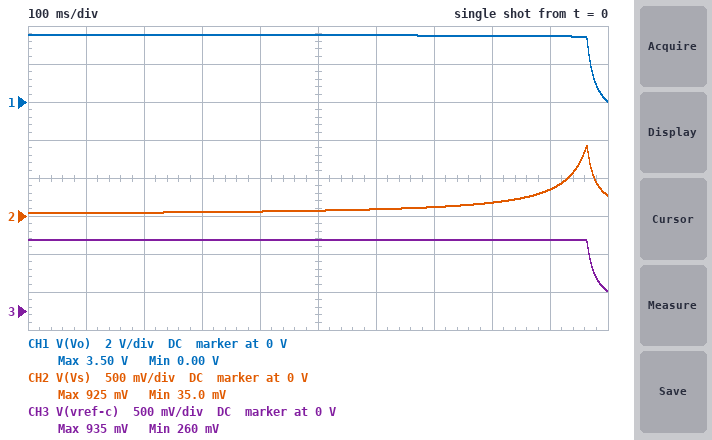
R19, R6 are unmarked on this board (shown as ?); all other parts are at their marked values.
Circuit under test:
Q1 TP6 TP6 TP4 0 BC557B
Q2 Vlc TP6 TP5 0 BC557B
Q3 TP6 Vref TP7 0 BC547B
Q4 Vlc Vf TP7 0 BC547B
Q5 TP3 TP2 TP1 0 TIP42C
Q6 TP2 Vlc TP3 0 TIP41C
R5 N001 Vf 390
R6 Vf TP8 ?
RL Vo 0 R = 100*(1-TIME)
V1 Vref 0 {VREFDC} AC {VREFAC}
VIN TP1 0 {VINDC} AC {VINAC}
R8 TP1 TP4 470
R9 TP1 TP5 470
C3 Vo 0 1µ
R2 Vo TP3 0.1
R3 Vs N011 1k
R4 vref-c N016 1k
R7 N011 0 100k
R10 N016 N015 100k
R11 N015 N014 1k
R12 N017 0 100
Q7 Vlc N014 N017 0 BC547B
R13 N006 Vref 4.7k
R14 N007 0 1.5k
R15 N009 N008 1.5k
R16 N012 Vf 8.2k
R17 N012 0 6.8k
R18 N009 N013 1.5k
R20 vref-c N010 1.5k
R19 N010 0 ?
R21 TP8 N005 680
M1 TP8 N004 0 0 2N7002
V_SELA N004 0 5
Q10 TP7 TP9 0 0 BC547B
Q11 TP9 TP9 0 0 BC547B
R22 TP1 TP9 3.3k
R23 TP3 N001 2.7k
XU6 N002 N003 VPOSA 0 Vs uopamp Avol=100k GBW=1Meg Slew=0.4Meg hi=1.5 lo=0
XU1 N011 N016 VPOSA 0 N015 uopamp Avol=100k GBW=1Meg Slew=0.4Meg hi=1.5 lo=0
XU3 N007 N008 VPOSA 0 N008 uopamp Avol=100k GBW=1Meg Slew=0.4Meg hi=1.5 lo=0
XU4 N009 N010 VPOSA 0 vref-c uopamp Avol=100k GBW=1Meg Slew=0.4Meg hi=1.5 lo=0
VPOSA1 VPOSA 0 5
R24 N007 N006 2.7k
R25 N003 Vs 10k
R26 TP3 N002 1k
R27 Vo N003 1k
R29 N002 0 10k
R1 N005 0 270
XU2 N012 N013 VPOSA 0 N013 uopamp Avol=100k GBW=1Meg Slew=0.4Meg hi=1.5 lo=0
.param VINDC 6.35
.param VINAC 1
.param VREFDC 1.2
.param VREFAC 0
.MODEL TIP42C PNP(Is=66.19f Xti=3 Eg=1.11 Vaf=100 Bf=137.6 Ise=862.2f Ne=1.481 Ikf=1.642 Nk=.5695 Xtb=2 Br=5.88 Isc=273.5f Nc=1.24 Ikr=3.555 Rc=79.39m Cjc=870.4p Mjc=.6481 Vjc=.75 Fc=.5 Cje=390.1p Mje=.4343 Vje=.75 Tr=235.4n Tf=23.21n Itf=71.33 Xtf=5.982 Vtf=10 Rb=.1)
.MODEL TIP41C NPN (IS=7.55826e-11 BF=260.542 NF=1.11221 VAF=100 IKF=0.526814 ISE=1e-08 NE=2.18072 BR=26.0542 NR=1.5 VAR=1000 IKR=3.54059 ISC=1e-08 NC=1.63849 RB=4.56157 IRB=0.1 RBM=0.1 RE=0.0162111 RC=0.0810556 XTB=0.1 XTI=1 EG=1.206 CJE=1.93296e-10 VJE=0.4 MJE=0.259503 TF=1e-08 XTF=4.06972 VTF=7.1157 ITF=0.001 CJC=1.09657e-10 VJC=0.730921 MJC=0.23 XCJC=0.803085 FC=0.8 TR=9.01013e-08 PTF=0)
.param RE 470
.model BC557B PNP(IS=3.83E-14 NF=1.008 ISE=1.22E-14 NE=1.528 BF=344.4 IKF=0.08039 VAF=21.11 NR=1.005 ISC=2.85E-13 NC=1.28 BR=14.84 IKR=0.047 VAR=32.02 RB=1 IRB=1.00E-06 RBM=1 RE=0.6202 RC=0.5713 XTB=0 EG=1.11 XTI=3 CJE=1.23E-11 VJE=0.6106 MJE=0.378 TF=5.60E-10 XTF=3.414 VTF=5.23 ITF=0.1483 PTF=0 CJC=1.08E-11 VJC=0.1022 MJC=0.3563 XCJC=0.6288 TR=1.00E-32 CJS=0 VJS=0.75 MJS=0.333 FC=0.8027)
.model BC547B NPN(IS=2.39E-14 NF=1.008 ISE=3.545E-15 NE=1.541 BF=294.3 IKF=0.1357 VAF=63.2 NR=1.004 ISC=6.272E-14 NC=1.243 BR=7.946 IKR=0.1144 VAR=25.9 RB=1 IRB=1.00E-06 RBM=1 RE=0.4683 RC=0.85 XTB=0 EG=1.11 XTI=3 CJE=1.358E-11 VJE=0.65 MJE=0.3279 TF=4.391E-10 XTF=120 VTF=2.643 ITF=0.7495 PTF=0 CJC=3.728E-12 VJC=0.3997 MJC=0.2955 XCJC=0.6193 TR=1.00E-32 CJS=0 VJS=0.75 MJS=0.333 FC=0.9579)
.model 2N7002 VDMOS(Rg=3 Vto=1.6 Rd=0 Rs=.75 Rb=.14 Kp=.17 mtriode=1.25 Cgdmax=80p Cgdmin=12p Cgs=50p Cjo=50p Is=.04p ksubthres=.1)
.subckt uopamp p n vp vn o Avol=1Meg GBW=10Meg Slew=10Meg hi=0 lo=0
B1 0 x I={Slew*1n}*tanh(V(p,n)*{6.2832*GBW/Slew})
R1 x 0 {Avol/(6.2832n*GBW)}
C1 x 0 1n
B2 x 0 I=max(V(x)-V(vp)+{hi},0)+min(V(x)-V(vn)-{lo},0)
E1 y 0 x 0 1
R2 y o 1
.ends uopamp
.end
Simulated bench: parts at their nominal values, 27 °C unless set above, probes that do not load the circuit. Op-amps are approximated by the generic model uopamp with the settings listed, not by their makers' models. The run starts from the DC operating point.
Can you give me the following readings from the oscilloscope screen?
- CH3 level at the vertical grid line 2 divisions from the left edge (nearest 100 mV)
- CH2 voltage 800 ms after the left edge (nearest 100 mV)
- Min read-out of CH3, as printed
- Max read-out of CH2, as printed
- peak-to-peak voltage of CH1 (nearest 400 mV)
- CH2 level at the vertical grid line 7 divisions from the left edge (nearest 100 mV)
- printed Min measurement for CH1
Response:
900 mV
200 mV
260 mV
925 mV
3.6 V
100 mV
0.00 V
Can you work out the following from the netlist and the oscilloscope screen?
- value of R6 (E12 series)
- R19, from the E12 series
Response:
1.8 kΩ
1 kΩ
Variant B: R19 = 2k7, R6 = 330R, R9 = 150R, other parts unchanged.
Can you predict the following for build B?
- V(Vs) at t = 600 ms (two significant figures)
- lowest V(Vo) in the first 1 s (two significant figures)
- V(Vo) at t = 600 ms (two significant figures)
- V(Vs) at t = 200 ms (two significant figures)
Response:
140 mV
-16 mV
5.6 V
71 mV
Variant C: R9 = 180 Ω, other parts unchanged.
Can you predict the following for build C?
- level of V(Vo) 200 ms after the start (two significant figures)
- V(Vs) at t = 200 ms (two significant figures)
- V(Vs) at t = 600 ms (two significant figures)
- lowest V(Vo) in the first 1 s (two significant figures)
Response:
3.6 V
45 mV
90 mV
-2.7 mV
